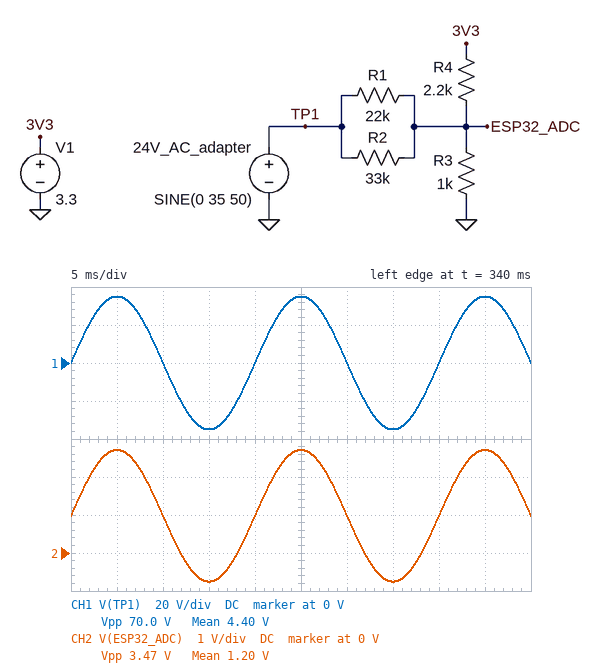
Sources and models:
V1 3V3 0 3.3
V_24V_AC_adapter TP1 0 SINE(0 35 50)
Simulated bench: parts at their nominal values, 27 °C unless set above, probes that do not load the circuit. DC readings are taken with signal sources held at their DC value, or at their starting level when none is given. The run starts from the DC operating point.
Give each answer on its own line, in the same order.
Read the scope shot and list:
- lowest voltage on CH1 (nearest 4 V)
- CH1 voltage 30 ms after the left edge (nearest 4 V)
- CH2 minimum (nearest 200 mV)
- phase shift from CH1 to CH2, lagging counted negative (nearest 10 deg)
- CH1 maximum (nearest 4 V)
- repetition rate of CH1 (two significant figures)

-36 V
0 V
-800 mV
0 deg
36 V
50 Hz
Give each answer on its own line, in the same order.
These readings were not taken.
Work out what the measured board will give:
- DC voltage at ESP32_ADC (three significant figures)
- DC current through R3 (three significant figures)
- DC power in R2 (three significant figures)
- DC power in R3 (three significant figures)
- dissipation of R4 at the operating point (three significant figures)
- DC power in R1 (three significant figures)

980 mV
980 µA
29.1 µW
961 µW
2.45 mW
43.7 µW
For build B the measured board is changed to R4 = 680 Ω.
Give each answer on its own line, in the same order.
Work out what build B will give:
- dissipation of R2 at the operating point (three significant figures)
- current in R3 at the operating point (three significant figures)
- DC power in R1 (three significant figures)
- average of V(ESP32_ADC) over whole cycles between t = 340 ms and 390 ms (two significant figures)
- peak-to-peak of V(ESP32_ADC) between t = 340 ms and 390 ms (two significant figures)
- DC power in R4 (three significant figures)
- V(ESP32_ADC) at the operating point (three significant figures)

110 µW
1.91 mA
165 µW
1.9 V
2.1 V
2.86 mW
1.91 V
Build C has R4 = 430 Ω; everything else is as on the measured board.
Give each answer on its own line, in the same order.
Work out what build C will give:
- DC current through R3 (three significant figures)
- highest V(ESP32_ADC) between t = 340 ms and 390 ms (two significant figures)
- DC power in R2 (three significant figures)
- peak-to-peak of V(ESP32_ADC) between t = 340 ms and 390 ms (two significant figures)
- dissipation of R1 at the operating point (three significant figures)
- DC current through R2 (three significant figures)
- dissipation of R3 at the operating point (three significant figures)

2.26 mA
3.0 V
154 µW
1.6 V
231 µW
68.4 µA
5.09 mW
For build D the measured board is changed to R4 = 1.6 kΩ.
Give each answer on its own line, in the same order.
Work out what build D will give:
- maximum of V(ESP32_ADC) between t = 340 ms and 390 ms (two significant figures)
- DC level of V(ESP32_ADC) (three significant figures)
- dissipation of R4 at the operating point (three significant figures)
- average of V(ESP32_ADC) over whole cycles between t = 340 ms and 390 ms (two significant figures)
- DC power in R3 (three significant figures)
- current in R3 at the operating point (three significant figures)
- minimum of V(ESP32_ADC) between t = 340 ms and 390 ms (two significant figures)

2.8 V
1.21 V
2.72 mW
1.2 V
1.47 mW
1.21 mA
-350 mV
